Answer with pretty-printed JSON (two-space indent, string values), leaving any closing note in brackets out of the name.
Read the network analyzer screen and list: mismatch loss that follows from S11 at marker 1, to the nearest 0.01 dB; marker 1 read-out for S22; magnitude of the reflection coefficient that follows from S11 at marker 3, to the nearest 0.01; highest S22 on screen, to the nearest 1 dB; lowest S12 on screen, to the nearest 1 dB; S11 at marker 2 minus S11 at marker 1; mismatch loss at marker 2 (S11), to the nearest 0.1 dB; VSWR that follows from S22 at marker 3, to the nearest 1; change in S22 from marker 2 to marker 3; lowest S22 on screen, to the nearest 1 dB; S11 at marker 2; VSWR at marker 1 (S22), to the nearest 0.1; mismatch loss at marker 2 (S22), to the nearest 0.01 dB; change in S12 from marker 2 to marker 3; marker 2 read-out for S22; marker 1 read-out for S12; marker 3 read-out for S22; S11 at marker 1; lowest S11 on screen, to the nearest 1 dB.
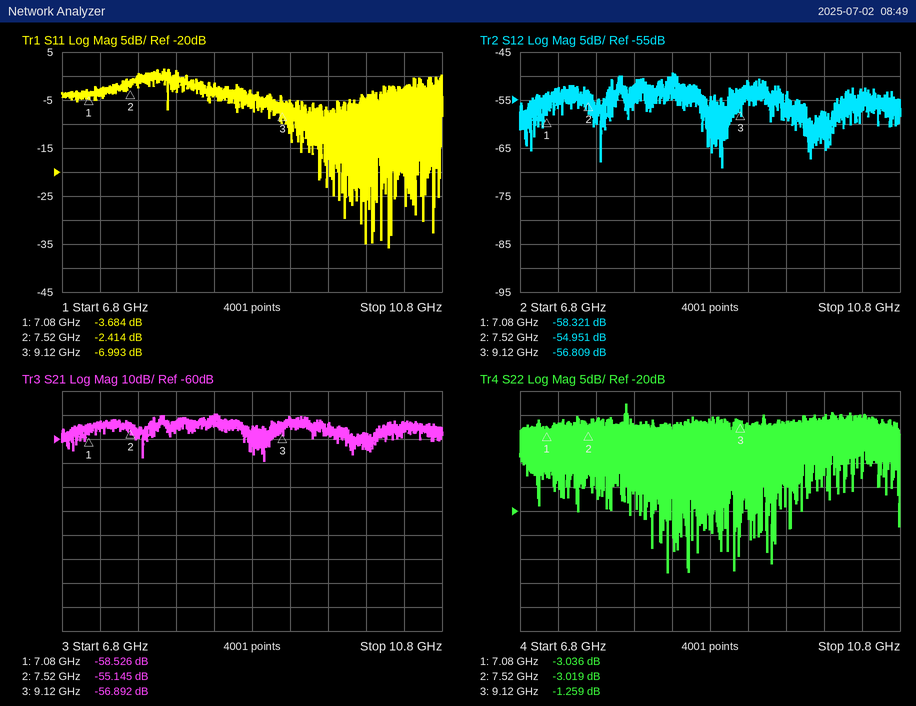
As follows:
{
  "mismatch loss that follows from S11 at marker 1, to the nearest 0.01 dB": "2.43 dB",
  "marker 1 read-out for S22": "-3.036 dB",
  "magnitude of the reflection coefficient that follows from S11 at marker 3, to the nearest 0.01": "0.45",
  "highest S22 on screen, to the nearest 1 dB": "2 dB",
  "lowest S12 on screen, to the nearest 1 dB": "-69 dB",
  "S11 at marker 2 minus S11 at marker 1": "1.270 dB",
  "mismatch loss at marker 2 (S11), to the nearest 0.1 dB": "3.7 dB",
  "VSWR that follows from S22 at marker 3, to the nearest 1": "14",
  "change in S22 from marker 2 to marker 3": "1.760 dB",
  "lowest S22 on screen, to the nearest 1 dB": "-33 dB",
  "S11 at marker 2": "-2.414 dB",
  "VSWR at marker 1 (S22), to the nearest 0.1": "5.8",
  "mismatch loss at marker 2 (S22), to the nearest 0.01 dB": "3.00 dB",
  "change in S12 from marker 2 to marker 3": "-1.858 dB",
  "marker 2 read-out for S22": "-3.019 dB",
  "marker 1 read-out for S12": "-58.321 dB",
  "marker 3 read-out for S22": "-1.259 dB",
  "S11 at marker 1": "-3.684 dB",
  "lowest S11 on screen, to the nearest 1 dB": "-36 dB"
}
